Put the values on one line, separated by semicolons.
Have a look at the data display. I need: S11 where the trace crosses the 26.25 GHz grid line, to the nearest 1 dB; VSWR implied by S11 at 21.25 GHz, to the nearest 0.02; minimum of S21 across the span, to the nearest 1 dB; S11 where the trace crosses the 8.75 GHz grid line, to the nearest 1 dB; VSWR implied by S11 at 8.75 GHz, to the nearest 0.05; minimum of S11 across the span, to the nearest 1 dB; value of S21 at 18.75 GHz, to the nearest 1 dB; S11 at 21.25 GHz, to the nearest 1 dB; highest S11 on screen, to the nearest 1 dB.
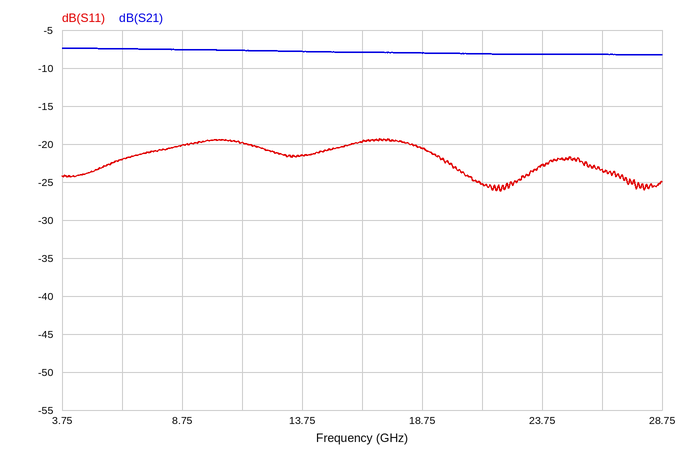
-23 dB; 1.12; -8 dB; -20 dB; 1.20; -26 dB; -8 dB; -25 dB; -19 dB
